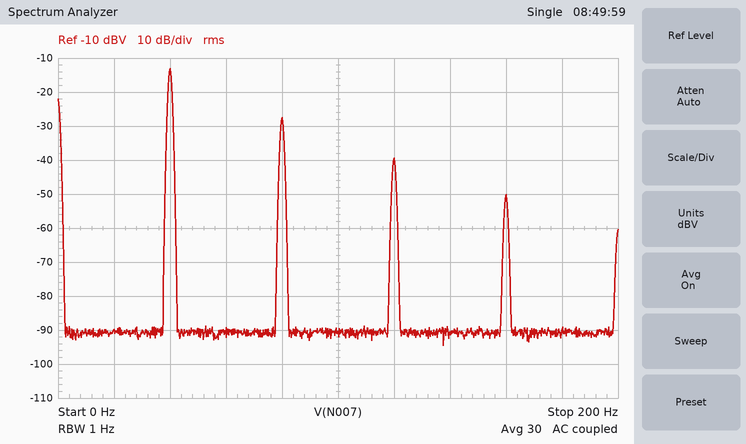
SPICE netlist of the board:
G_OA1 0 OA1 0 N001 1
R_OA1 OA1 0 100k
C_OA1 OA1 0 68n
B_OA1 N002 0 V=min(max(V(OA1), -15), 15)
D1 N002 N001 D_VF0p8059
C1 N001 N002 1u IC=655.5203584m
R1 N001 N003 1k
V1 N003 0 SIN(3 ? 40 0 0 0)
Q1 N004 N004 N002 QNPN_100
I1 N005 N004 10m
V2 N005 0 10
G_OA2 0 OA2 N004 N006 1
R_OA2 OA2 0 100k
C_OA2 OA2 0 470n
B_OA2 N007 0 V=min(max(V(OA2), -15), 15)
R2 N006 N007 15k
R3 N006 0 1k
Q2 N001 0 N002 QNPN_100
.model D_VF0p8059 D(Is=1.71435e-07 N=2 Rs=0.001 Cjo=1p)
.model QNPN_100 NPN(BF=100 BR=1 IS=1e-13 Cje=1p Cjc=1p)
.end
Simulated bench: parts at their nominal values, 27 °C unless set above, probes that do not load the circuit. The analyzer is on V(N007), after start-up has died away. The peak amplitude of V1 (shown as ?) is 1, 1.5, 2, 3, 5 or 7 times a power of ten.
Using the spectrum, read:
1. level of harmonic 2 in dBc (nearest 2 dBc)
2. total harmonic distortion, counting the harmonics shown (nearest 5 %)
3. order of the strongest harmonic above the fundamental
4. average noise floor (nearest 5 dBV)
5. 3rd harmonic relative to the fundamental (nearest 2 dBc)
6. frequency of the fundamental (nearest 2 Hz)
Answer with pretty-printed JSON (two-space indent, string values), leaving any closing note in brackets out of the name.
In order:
{
  "level of harmonic 2 in dBc": "-14 dBc",
  "total harmonic distortion, counting the harmonics shown": "20 %",
  "order of the strongest harmonic above the fundamental": "2",
  "average noise floor": "-90 dBV",
  "3rd harmonic relative to the fundamental": "-26 dBc",
  "frequency of the fundamental": "40 Hz"
}
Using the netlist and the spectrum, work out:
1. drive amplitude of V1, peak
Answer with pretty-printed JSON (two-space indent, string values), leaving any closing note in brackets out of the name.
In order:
{
  "drive amplitude of V1, peak": "2 V"
}
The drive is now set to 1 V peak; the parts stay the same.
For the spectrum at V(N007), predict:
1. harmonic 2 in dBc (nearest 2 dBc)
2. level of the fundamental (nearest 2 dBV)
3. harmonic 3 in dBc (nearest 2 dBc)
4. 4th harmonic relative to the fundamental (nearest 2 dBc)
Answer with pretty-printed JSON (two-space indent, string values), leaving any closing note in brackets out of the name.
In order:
{
  "harmonic 2 in dBc": "-22 dBc",
  "level of the fundamental": "-20 dBV",
  "harmonic 3 in dBc": "-40 dBc",
  "4th harmonic relative to the fundamental": "-58 dBc"
}
